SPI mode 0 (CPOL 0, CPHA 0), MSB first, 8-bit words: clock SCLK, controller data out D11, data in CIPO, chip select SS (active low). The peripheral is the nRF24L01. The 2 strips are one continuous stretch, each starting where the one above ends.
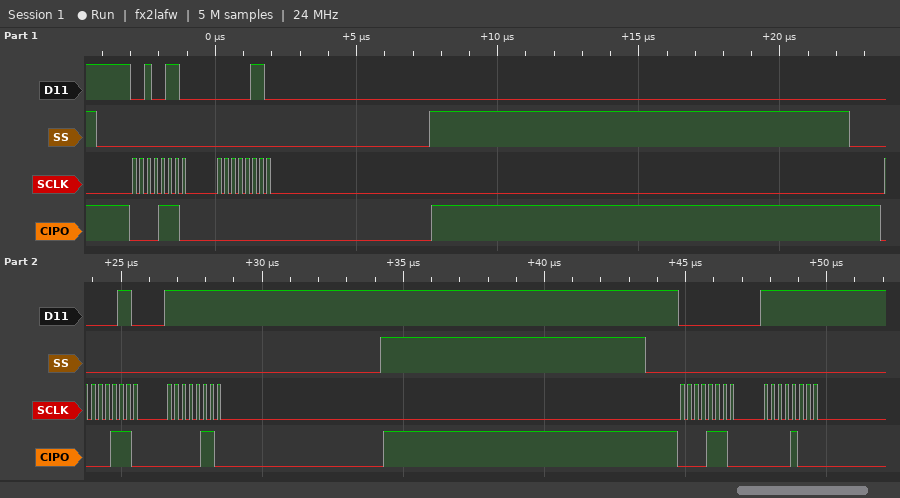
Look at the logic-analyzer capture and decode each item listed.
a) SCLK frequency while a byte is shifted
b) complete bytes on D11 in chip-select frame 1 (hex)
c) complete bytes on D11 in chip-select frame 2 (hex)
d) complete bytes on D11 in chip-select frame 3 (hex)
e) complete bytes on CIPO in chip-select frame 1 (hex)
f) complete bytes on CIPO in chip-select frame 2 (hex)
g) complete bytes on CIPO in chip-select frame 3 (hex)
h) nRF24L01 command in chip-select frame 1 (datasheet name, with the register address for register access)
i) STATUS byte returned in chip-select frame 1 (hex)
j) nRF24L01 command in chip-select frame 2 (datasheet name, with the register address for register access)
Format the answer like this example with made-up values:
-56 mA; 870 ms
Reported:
4 MHz; 0x26 0x06; 0x06 0xFF; 0x00 0xFF; 0x0E 0x00; 0x0E 0x06; 0x0E 0x08; W_REGISTER 0x06; 0x0E; R_REGISTER 0x06
